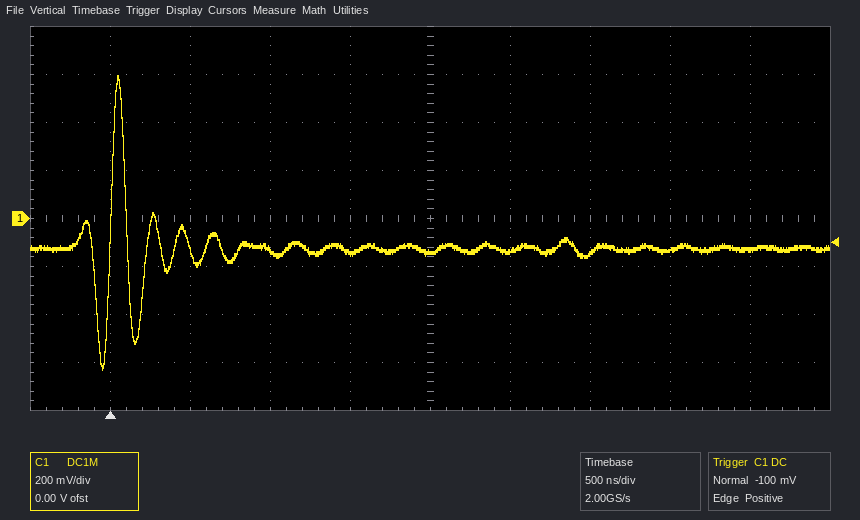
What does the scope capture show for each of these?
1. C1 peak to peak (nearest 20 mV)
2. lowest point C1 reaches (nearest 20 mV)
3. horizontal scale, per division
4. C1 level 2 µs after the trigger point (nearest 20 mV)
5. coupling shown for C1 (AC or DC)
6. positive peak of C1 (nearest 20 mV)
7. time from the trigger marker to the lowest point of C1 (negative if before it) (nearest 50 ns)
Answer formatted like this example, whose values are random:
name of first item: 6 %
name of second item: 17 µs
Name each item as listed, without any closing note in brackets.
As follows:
C1 peak to peak: 1.22 V
lowest point C1 reaches: -620 mV
horizontal scale, per division: 500 ns
C1 level 2 µs after the trigger point: -140 mV
coupling shown for C1: DC
positive peak of C1: 600 mV
time from the trigger marker to the lowest point of C1 (negative if before it): -50 ns
